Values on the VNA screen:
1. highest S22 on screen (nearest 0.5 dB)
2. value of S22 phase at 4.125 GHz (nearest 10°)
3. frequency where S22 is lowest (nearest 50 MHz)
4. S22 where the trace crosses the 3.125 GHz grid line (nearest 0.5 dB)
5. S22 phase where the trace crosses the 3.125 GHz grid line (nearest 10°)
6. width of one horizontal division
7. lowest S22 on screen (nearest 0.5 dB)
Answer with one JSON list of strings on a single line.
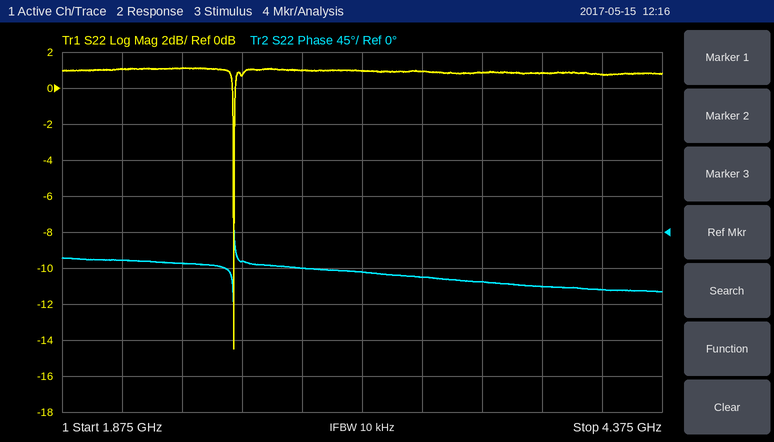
["1.0 dB", "-70°", "2.60 GHz", "1.0 dB", "-50°", "250 MHz", "-14.5 dB"]
